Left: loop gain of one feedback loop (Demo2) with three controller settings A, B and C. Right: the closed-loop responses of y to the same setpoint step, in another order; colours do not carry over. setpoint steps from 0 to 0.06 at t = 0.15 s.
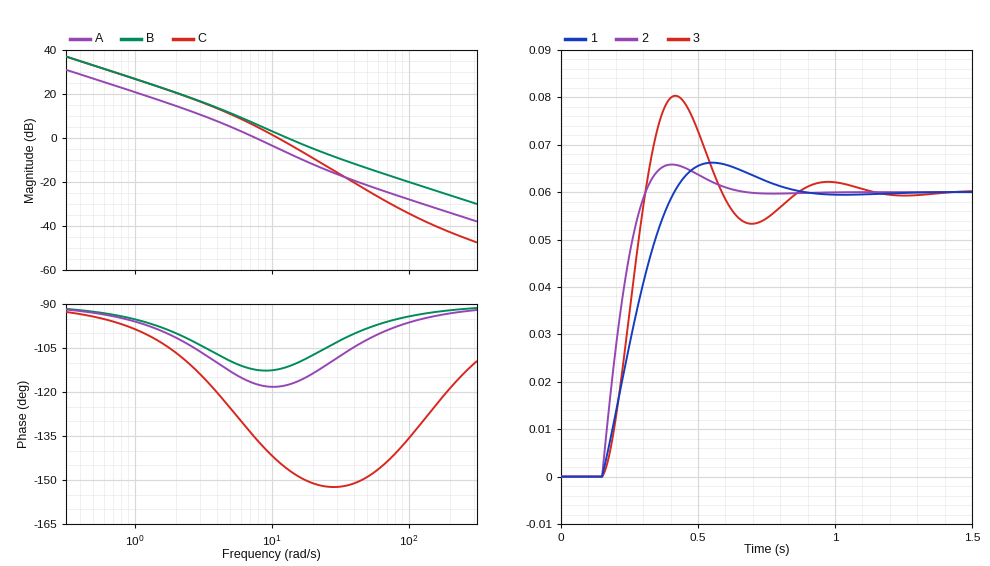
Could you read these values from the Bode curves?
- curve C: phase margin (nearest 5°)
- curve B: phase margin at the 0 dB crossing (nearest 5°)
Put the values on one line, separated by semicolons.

35°; 70°
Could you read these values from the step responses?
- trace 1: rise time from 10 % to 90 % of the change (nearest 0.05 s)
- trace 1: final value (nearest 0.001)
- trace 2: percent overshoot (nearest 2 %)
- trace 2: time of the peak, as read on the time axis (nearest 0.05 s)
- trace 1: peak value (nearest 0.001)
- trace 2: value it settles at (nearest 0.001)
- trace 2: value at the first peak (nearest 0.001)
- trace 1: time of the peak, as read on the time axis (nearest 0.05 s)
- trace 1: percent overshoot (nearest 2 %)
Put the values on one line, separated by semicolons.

0.20 s; 0.060; 10 %; 0.40 s; 0.066; 0.060; 0.066; 0.55 s; 10 %
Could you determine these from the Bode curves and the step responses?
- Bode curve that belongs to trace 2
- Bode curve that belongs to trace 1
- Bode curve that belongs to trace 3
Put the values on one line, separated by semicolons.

B; A; C
